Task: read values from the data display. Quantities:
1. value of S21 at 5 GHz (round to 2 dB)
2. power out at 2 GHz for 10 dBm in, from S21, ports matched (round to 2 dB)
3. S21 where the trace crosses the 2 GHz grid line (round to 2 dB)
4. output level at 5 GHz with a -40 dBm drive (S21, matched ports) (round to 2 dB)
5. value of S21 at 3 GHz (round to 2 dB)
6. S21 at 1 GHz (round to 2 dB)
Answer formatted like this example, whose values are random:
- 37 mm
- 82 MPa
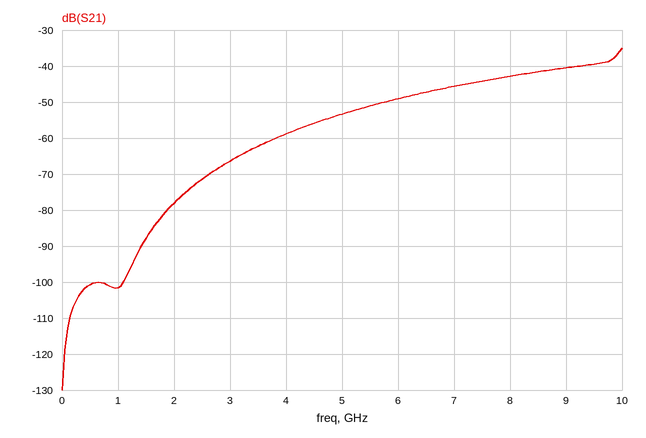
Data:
- -54 dB
- -68 dBm
- -78 dB
- -94 dBm
- -66 dB
- -102 dB
